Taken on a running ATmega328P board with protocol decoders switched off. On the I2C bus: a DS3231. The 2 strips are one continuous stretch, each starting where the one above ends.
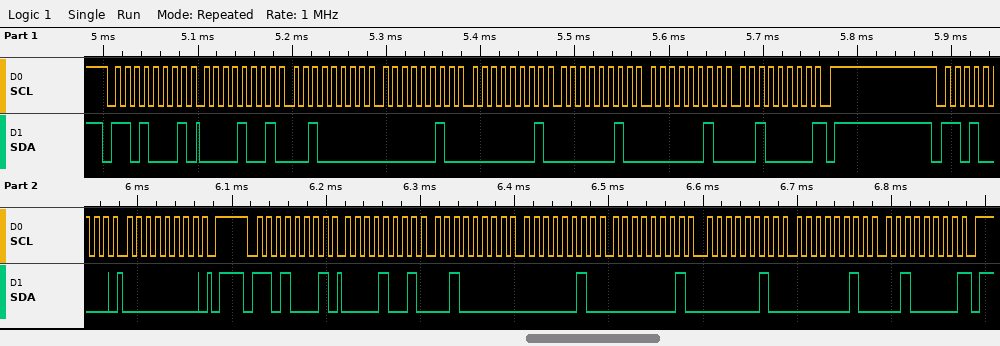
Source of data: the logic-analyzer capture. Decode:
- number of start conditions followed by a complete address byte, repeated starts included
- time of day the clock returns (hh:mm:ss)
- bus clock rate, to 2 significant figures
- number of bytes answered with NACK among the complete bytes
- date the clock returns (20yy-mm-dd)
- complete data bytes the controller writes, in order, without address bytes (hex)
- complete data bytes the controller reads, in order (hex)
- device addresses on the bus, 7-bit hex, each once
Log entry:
3
02:20:09
100 kHz
2
2020-02-02
00
09 20 02 01 02 02 20 09 20 02 01 02 02 20
0x68
